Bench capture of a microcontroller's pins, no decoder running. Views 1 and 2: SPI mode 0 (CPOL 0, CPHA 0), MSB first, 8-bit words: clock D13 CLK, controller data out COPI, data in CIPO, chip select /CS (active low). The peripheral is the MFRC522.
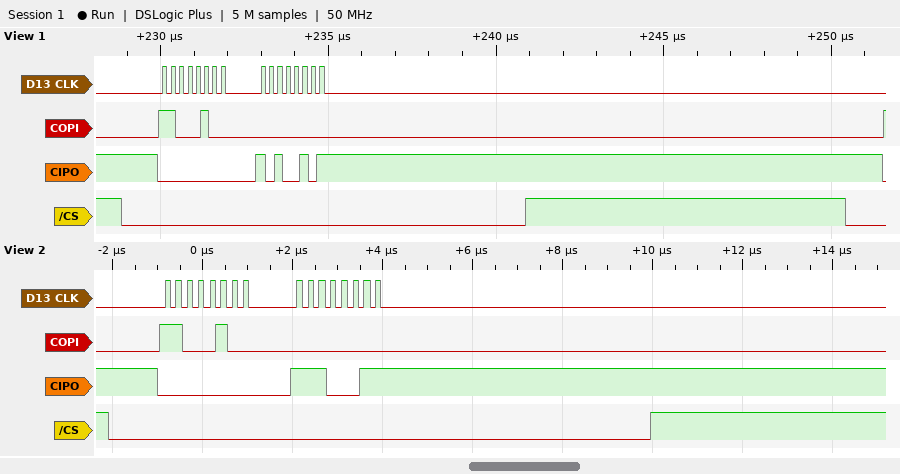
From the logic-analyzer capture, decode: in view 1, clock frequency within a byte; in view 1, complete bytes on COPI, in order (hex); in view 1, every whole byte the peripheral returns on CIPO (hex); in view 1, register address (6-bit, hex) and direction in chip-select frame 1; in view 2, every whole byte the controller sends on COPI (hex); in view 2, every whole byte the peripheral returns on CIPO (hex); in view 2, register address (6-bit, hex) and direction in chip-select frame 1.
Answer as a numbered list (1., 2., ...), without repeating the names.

1. 4 MHz
2. C4 00
3. 00 A5
4. 0x22 read
5. 0xC4 0x00
6. 0x00 0xE3
7. 0x22 read
